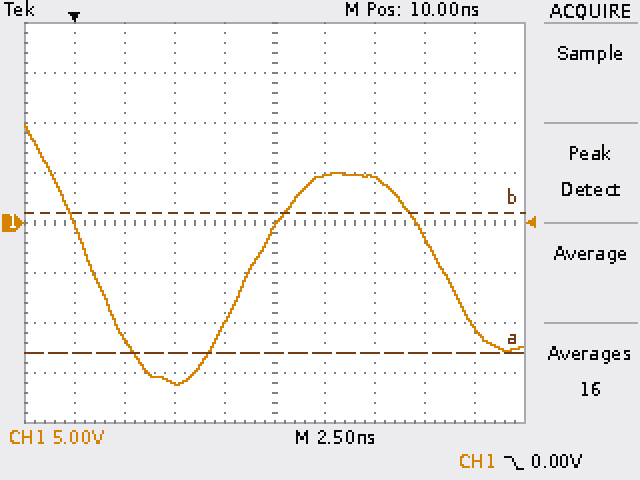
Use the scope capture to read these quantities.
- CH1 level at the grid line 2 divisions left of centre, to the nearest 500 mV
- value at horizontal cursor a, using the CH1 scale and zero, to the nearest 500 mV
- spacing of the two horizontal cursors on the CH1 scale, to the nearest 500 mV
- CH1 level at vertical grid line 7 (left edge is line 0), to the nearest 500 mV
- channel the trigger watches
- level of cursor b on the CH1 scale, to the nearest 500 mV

-16.0 V
-13.0 V
14.0 V
4.5 V
CH1
1.0 V
